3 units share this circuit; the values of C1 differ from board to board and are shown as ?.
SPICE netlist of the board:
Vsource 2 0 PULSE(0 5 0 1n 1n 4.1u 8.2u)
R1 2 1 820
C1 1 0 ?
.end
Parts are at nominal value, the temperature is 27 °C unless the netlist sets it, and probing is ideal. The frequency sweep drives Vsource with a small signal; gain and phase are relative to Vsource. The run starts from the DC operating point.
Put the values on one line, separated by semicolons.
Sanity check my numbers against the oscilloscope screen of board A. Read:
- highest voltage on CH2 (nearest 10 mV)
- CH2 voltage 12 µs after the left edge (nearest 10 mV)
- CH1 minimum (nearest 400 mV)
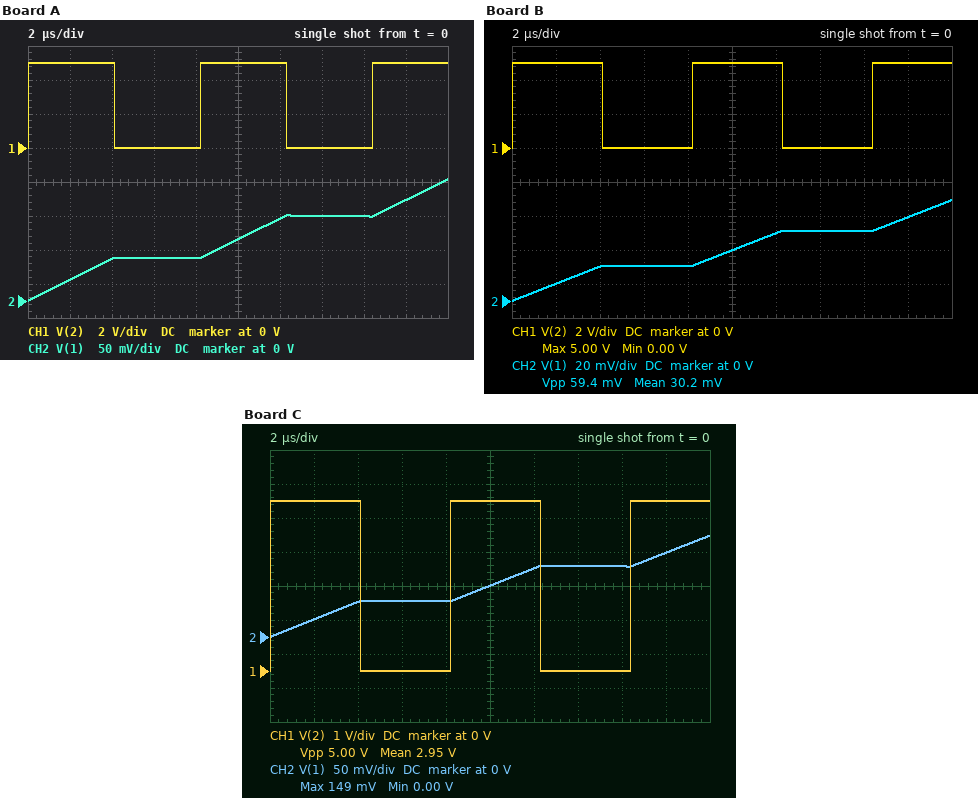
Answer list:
180 mV; 120 mV; 0 V
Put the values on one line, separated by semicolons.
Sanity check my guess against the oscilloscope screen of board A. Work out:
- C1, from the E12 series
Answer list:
390 nF
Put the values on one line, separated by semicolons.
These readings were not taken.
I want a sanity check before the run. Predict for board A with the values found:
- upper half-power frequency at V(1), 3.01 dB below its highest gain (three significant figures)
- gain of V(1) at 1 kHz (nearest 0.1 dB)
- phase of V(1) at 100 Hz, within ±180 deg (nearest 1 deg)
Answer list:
498 Hz; -7.0 dB; -11 deg
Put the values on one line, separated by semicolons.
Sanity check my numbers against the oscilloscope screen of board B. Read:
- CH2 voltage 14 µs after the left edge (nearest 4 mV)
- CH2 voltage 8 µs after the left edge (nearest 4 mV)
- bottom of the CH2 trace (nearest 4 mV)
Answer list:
40 mV; 20 mV; 0 V
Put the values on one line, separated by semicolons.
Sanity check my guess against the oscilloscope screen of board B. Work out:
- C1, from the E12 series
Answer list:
1.2 µF
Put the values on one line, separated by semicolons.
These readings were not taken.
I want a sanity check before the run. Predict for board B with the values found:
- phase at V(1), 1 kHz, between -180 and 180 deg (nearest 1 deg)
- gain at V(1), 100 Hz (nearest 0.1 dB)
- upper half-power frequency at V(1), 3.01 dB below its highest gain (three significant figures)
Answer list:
-81 deg; -1.4 dB; 162 Hz
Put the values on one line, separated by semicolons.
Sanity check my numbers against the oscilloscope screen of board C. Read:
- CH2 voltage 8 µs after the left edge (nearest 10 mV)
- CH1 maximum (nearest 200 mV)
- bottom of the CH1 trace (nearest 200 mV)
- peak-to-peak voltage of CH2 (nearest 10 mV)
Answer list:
50 mV; 5.0 V; 0 V; 150 mV
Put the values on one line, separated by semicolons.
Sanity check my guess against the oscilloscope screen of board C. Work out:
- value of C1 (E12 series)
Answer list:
470 nF
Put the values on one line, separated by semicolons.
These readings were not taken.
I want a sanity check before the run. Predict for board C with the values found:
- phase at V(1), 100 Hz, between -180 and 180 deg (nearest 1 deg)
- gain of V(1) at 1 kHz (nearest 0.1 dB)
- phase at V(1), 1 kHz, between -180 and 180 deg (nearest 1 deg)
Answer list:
-14 deg; -8.4 dB; -68 deg
